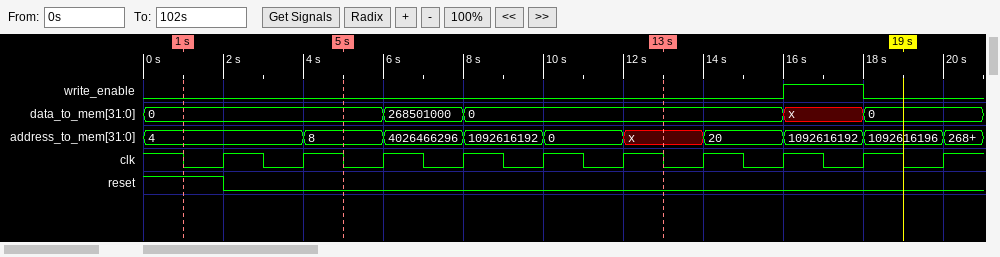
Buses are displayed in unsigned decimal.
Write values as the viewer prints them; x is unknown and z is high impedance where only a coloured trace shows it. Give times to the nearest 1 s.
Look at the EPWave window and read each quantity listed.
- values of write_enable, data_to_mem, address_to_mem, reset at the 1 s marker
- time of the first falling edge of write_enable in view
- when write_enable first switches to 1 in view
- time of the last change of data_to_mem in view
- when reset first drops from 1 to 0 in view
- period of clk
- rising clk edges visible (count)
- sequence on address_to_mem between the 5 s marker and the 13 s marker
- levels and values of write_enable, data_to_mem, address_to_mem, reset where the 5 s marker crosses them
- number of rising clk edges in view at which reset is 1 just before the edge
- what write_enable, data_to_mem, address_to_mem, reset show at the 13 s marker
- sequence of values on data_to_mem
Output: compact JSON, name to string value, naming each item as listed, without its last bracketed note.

{"values of write_enable, data_to_mem, address_to_mem, reset at the 1 s marker": "write_enable=0, data_to_mem=0, address_to_mem=4, reset=1", "time of the first falling edge of write_enable in view": "18 s", "when write_enable first switches to 1 in view": "16 s", "time of the last change of data_to_mem in view": "18 s", "when reset first drops from 1 to 0 in view": "2 s", "period of clk": "2 s", "rising clk edges visible": "10", "sequence on address_to_mem between the 5 s marker and the 13 s marker": "8, 4026466296, 1092616192, 0, x", "levels and values of write_enable, data_to_mem, address_to_mem, reset where the 5 s marker crosses them": "write_enable=0, data_to_mem=0, address_to_mem=8, reset=0", "number of rising clk edges in view at which reset is 1 just before the edge": "1", "what write_enable, data_to_mem, address_to_mem, reset show at the 13 s marker": "write_enable=0, data_to_mem=0, address_to_mem=x, reset=0", "sequence of values on data_to_mem": "0, 268501000, 0, x, 0"}
